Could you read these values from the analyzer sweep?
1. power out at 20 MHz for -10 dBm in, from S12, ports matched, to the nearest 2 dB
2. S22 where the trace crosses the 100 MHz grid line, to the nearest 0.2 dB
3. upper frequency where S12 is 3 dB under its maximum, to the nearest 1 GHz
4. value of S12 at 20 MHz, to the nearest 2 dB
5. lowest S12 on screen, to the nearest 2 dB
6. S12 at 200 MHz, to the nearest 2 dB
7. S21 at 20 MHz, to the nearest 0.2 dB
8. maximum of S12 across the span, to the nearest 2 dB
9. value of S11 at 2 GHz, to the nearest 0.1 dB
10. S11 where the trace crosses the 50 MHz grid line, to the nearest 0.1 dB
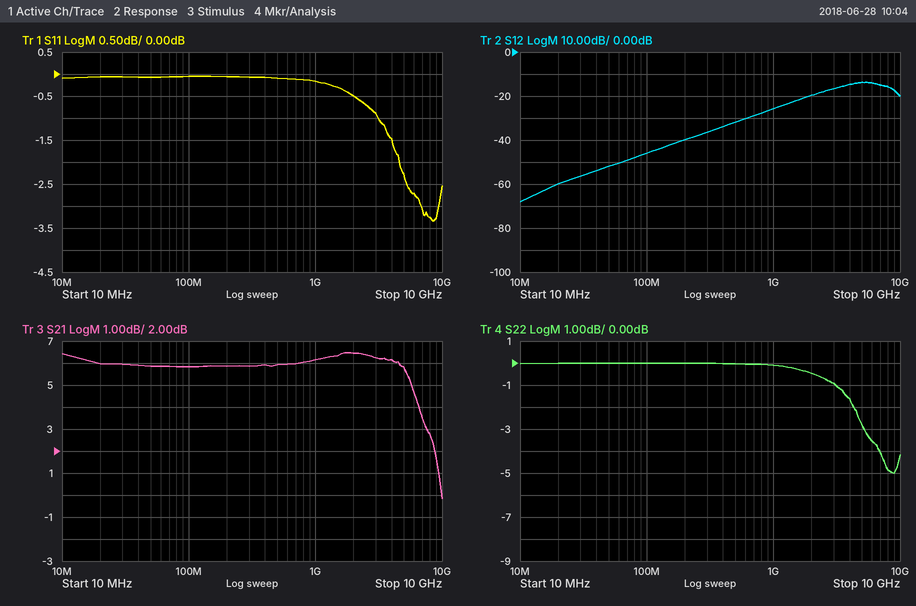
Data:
-70 dBm
0.0 dB
9 GHz
-60 dB
-68 dB
-40 dB
6.0 dB
-14 dB
-0.5 dB
-0.1 dB
